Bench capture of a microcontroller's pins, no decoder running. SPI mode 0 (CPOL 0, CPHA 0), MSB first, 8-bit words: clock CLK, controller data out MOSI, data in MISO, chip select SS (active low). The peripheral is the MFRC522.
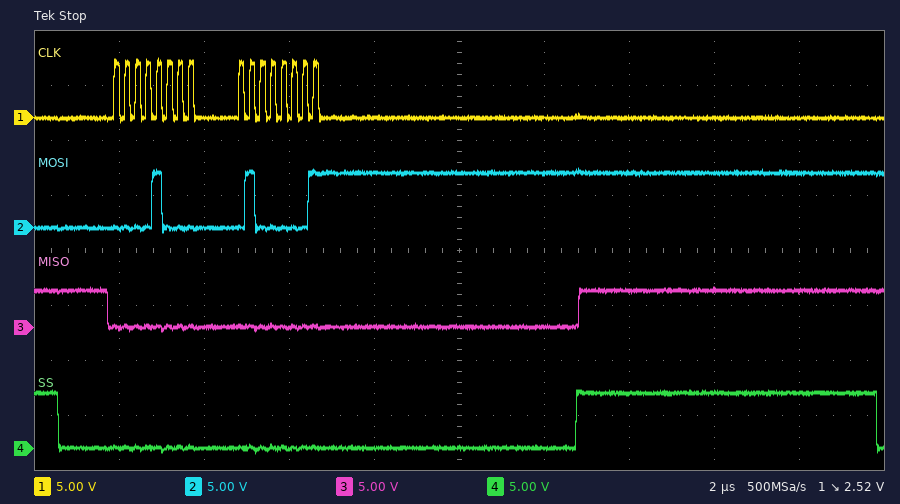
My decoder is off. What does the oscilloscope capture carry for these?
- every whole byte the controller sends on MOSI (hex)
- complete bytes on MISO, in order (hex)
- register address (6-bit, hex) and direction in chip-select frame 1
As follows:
0x08 0x41
0x00 0x00
0x04 write
